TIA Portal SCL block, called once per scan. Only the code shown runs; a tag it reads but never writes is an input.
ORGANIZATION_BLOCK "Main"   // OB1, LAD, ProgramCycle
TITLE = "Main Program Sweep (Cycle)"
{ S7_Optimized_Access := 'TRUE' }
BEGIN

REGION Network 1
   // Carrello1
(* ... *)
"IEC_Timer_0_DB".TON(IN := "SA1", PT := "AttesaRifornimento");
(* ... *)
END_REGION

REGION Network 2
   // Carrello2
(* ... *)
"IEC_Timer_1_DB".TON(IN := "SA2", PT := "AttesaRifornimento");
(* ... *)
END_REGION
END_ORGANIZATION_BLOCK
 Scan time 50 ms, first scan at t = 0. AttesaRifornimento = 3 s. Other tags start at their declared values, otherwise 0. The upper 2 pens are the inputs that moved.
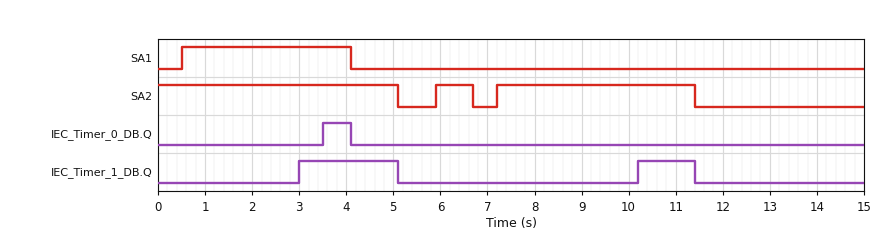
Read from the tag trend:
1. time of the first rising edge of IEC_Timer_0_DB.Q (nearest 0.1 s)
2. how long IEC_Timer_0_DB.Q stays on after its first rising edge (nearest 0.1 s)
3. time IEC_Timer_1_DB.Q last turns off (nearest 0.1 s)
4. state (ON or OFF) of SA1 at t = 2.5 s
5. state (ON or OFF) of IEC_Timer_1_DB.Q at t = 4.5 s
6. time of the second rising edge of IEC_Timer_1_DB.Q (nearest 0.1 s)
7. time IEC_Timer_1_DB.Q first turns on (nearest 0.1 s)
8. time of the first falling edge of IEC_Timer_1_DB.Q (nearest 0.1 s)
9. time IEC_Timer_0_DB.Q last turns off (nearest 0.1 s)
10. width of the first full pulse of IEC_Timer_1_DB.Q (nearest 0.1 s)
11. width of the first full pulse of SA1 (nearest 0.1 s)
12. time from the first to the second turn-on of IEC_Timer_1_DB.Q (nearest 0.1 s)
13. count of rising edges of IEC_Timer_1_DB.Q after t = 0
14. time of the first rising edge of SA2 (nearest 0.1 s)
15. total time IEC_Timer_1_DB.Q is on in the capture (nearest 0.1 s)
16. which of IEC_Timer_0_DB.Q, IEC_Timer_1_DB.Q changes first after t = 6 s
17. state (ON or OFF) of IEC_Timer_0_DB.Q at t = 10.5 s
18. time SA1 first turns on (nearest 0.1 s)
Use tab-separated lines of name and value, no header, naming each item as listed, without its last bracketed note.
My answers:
time of the first rising edge of IEC_Timer_0_DB.Q	3.5 s
how long IEC_Timer_0_DB.Q stays on after its first rising edge	0.6 s
time IEC_Timer_1_DB.Q last turns off	11.4 s
state (ON or OFF) of SA1 at t = 2.5 s	ON
state (ON or OFF) of IEC_Timer_1_DB.Q at t = 4.5 s	ON
time of the second rising edge of IEC_Timer_1_DB.Q	10.2 s
time IEC_Timer_1_DB.Q first turns on	3.0 s
time of the first falling edge of IEC_Timer_1_DB.Q	5.1 s
time IEC_Timer_0_DB.Q last turns off	4.1 s
width of the first full pulse of IEC_Timer_1_DB.Q	2.1 s
width of the first full pulse of SA1	3.6 s
time from the first to the second turn-on of IEC_Timer_1_DB.Q	7.2 s
count of rising edges of IEC_Timer_1_DB.Q after t = 0	2
time of the first rising edge of SA2	5.9 s
total time IEC_Timer_1_DB.Q is on in the capture	3.3 s
which of IEC_Timer_0_DB.Q, IEC_Timer_1_DB.Q changes first after t = 6 s	IEC_Timer_1_DB.Q
state (ON or OFF) of IEC_Timer_0_DB.Q at t = 10.5 s	OFF
time SA1 first turns on	0.5 s
